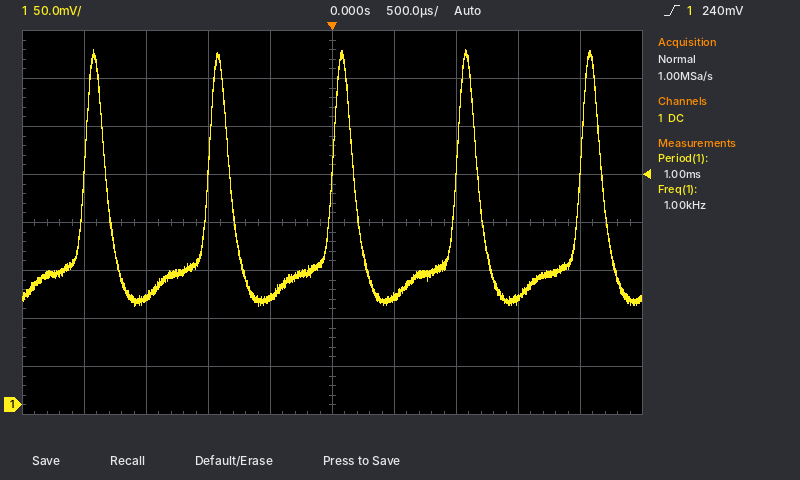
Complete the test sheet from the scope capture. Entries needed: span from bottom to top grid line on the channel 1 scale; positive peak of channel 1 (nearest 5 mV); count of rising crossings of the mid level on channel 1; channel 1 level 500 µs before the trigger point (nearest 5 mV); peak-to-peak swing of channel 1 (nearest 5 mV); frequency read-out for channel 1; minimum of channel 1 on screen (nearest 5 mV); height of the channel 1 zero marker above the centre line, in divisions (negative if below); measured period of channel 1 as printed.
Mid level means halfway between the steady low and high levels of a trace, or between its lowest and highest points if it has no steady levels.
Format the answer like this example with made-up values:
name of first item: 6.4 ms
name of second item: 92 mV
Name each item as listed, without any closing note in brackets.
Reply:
span from bottom to top grid line on the channel 1 scale: 400 mV
positive peak of channel 1: 370 mV
count of rising crossings of the mid level on channel 1: 5
channel 1 level 500 µs before the trigger point: 110 mV
peak-to-peak swing of channel 1: 265 mV
frequency read-out for channel 1: 1.00 kHz
minimum of channel 1 on screen: 105 mV
height of the channel 1 zero marker above the centre line, in divisions: -3.8 div
measured period of channel 1 as printed: 1.00 ms
